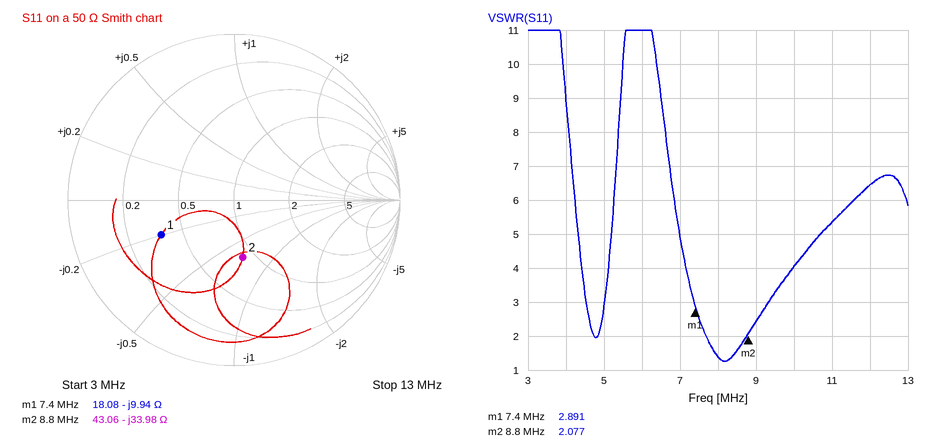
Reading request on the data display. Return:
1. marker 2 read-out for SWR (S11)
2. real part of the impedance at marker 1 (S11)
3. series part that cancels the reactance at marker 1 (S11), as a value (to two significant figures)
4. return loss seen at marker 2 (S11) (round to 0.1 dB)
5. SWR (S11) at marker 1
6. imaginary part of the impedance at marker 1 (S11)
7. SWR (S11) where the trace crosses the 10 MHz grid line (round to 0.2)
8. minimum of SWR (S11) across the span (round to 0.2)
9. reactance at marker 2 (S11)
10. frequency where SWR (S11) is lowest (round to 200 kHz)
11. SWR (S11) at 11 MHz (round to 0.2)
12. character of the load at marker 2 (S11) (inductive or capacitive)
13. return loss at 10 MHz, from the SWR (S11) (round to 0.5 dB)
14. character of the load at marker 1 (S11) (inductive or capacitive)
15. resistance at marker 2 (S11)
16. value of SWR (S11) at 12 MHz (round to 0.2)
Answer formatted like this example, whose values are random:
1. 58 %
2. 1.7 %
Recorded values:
1. 2.077
2. 18.08 Ω
3. 210 nH
4. 9.1 dB
5. 2.891
6. -9.94 Ω
7. 4.0
8. 1.2
9. -33.98 Ω
10. 8.2 MHz
11. 5.4
12. capacitive
13. 4.5 dB
14. capacitive
15. 43.06 Ω
16. 6.4
